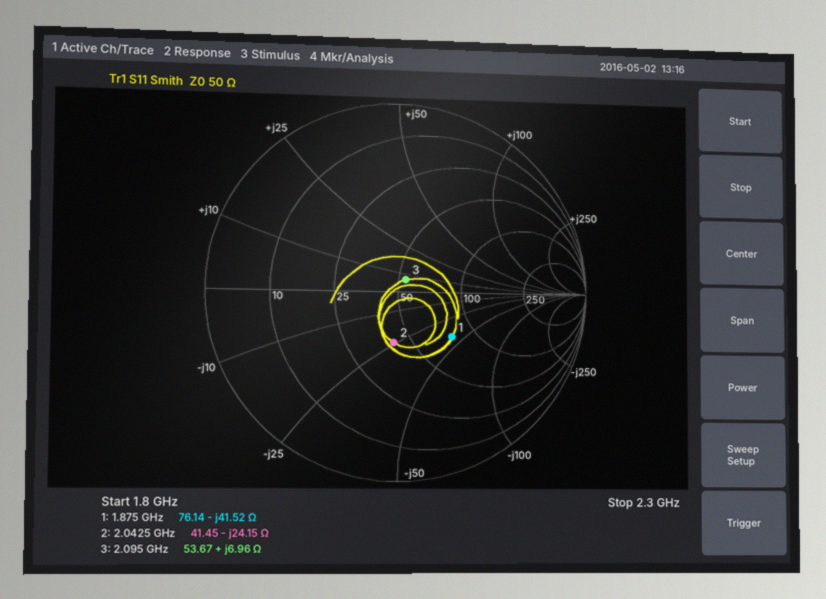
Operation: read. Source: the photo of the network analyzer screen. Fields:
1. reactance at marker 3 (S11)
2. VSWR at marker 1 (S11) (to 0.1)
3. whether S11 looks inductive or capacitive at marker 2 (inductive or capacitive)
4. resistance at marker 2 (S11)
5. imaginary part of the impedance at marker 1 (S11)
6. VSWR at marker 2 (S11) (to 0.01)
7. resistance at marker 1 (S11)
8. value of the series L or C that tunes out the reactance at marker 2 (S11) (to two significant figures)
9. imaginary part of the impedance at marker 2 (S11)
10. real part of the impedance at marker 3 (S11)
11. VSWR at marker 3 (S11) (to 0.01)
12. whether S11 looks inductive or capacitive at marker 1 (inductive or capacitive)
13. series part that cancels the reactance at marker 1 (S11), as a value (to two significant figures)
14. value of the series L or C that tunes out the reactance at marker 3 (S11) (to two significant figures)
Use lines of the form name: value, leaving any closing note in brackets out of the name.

reactance at marker 3: +6.96 Ω
VSWR at marker 1 (S11): 2.2
whether S11 looks inductive or capacitive at marker 2: capacitive
resistance at marker 2: 41.45 Ω
imaginary part of the impedance at marker 1: -41.52 Ω
VSWR at marker 2 (S11): 1.74
resistance at marker 1: 76.14 Ω
value of the series L or C that tunes out the reactance at marker 2 (S11): 1.9 nH
imaginary part of the impedance at marker 2: -24.15 Ω
real part of the impedance at marker 3: 53.67 Ω
VSWR at marker 3 (S11): 1.16
whether S11 looks inductive or capacitive at marker 1: capacitive
series part that cancels the reactance at marker 1 (S11), as a value: 3.5 nH
value of the series L or C that tunes out the reactance at marker 3 (S11): 11 pF
